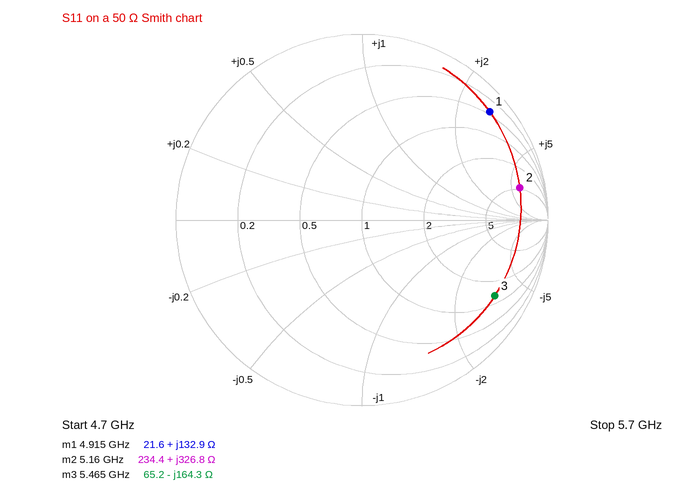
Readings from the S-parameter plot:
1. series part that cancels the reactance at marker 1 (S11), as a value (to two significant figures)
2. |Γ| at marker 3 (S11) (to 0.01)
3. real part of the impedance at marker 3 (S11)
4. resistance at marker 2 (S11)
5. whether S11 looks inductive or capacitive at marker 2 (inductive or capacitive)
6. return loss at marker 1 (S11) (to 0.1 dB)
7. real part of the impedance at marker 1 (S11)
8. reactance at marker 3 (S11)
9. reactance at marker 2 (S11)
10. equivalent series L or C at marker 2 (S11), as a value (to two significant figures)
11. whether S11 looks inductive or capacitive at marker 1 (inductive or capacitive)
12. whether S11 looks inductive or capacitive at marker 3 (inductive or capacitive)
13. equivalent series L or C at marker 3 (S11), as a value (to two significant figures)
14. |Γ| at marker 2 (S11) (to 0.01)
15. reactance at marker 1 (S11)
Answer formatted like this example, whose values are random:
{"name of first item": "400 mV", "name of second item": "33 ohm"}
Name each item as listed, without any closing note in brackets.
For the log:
{"series part that cancels the reactance at marker 1 (S11), as a value": "240 fF", "|Γ| at marker 3 (S11)": "0.82", "real part of the impedance at marker 3": "65.2 Ω", "resistance at marker 2": "234.4 Ω", "whether S11 looks inductive or capacitive at marker 2": "inductive", "return loss at marker 1 (S11)": "0.9 dB", "real part of the impedance at marker 1": "21.6 Ω", "reactance at marker 3": "-164.3 Ω", "reactance at marker 2": "+326.8 Ω", "equivalent series L or C at marker 2 (S11), as a value": "10 nH", "whether S11 looks inductive or capacitive at marker 1": "inductive", "whether S11 looks inductive or capacitive at marker 3": "capacitive", "equivalent series L or C at marker 3 (S11), as a value": "180 fF", "|Γ| at marker 2 (S11)": "0.87", "reactance at marker 1": "+132.9 Ω"}
